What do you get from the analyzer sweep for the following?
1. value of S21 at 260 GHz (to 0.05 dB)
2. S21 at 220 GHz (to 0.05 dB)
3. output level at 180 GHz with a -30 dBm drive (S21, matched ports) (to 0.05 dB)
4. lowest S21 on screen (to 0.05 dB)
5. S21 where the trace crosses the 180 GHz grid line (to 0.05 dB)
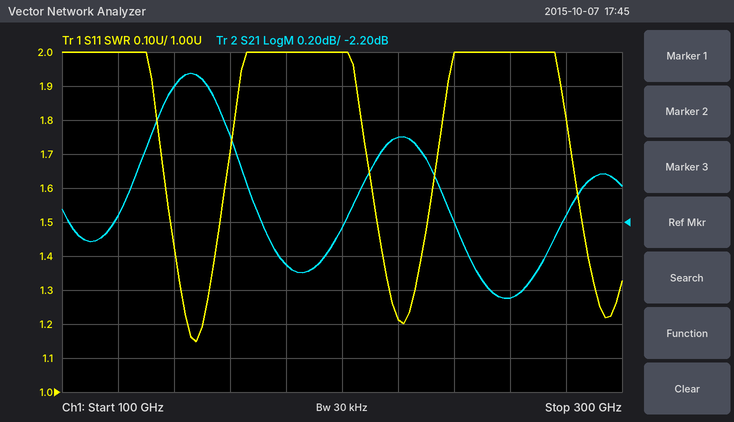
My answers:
-2.65 dB
-1.70 dB
-32.45 dBm
-2.65 dB
-2.45 dB
